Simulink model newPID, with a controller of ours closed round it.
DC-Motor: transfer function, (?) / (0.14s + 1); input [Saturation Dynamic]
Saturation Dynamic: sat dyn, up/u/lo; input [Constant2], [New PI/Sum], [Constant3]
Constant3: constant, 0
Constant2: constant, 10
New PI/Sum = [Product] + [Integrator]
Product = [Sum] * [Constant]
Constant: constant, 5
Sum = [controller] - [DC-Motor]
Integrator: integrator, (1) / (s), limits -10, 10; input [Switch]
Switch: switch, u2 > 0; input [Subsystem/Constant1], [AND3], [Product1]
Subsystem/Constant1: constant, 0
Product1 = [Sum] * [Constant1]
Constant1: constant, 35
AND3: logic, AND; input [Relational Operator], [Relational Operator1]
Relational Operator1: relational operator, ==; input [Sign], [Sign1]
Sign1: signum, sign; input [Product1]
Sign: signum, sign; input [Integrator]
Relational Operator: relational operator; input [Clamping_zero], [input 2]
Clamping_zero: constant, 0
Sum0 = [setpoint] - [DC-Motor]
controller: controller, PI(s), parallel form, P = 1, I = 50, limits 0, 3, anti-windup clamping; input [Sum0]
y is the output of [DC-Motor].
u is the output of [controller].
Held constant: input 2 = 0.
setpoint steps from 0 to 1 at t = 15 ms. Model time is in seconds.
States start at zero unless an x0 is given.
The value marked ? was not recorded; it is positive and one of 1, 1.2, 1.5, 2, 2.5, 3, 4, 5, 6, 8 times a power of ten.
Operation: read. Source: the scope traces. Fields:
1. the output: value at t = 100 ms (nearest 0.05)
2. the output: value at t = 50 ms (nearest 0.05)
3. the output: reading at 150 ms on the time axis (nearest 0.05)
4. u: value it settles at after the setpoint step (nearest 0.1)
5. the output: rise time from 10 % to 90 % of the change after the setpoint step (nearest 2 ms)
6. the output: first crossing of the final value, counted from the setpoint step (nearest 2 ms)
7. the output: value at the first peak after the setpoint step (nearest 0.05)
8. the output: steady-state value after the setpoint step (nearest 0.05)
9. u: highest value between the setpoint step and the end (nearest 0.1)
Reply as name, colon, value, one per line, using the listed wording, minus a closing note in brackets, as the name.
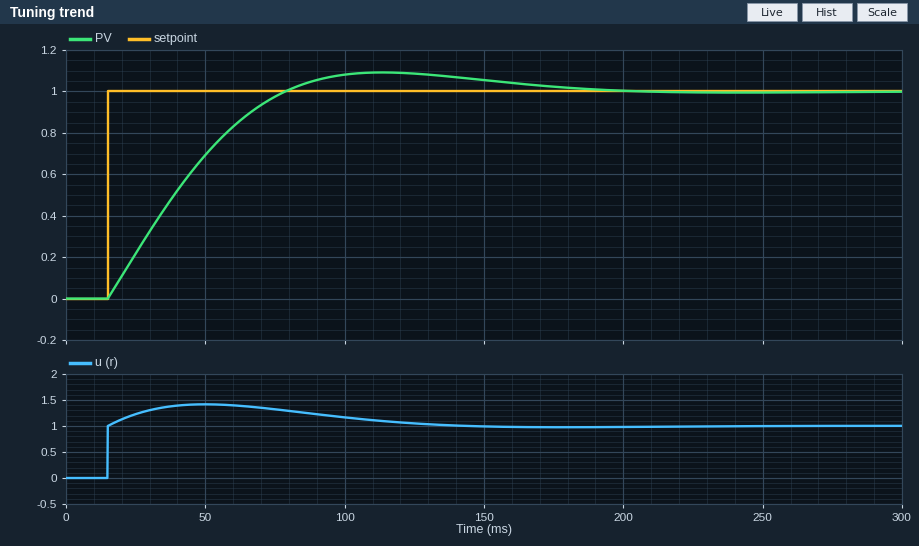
the output: value at t = 100 ms: 1.10
the output: value at t = 50 ms: 0.70
the output: reading at 150 ms on the time axis: 1.05
u: value it settles at after the setpoint step: 1.0
the output: rise time from 10 % to 90 % of the change after the setpoint step: 46 ms
the output: first crossing of the final value, counted from the setpoint step: 64 ms
the output: value at the first peak after the setpoint step: 1.10
the output: steady-state value after the setpoint step: 1.00
u: highest value between the setpoint step and the end: 1.4
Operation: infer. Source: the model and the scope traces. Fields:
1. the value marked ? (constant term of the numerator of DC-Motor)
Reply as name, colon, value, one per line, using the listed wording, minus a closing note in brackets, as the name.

the value marked ?: 0.6
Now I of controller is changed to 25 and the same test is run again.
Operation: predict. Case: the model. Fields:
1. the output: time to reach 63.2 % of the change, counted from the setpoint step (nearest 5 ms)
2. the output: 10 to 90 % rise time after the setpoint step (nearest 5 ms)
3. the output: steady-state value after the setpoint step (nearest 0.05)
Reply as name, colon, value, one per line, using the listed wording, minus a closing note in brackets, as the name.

the output: time to reach 63.2 % of the change, counted from the setpoint step: 45 ms
the output: 10 to 90 % rise time after the setpoint step: 85 ms
the output: steady-state value after the setpoint step: 1.00
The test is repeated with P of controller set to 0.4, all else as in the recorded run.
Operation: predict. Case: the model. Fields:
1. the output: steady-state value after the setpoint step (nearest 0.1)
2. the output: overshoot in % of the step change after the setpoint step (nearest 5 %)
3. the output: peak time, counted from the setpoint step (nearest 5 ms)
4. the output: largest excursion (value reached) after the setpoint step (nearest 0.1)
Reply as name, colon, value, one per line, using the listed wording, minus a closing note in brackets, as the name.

the output: steady-state value after the setpoint step: 1.0
the output: overshoot in % of the step change after the setpoint step: 20 %
the output: peak time, counted from the setpoint step: 100 ms
the output: largest excursion (value reached) after the setpoint step: 1.2
